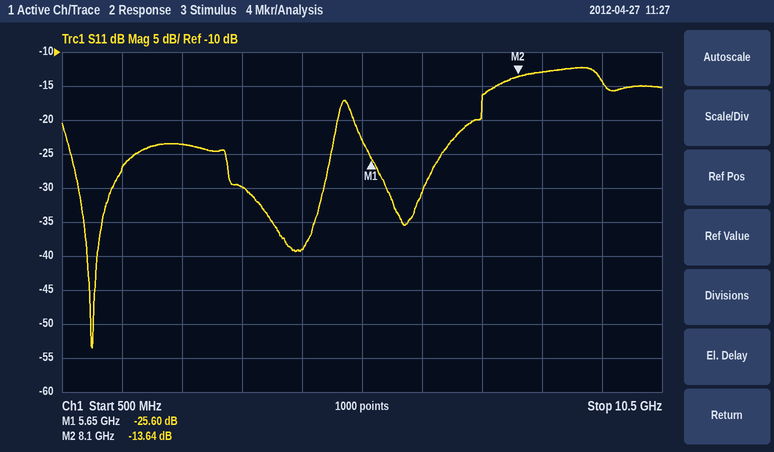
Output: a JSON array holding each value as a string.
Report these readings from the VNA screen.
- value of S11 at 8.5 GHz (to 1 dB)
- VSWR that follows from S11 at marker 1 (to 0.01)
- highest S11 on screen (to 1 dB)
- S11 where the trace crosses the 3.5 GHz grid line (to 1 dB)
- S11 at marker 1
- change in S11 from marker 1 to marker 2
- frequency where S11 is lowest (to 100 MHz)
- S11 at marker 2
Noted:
["-13 dB", "1.11", "-12 dB", "-30 dB", "-25.60 dB", "11.96 dB", "1.0 GHz", "-13.64 dB"]
